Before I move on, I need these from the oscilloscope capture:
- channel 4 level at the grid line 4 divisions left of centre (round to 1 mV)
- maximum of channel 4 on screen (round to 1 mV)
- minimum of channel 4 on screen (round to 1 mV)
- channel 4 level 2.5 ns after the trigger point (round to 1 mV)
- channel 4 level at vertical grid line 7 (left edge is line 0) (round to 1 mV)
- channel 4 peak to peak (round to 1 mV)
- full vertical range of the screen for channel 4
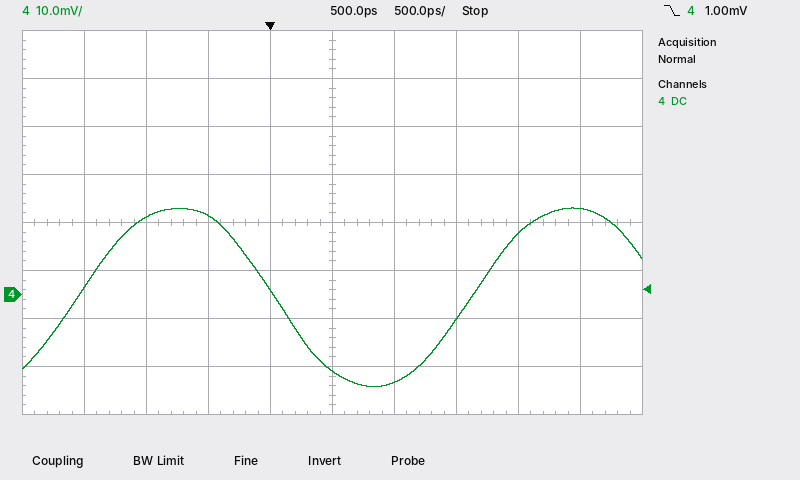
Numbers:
1 mV
18 mV
-19 mV
18 mV
-5 mV
37 mV
80 mV
